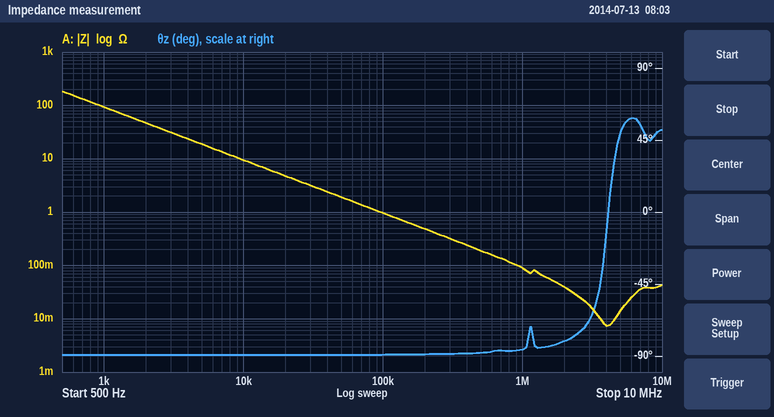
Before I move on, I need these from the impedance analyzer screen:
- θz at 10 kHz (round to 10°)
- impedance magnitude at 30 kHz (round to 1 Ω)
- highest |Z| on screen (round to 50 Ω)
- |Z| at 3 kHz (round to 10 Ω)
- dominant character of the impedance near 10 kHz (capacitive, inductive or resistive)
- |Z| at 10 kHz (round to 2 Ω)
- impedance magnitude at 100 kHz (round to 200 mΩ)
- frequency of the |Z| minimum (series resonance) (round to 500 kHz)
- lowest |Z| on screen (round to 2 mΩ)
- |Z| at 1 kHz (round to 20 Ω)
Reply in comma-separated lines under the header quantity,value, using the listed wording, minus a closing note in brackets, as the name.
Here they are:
quantity,value
θz at 10 kHz,-90°
impedance magnitude at 30 kHz,3 Ω
highest |Z| on screen,200 Ω
|Z| at 3 kHz,30 Ω
dominant character of the impedance near 10 kHz,capacitive
|Z| at 10 kHz,10 Ω
impedance magnitude at 100 kHz,1.0 Ω
frequency of the |Z| minimum (series resonance),4.0 MHz
lowest |Z| on screen,8 mΩ
|Z| at 1 kHz,100 Ω
